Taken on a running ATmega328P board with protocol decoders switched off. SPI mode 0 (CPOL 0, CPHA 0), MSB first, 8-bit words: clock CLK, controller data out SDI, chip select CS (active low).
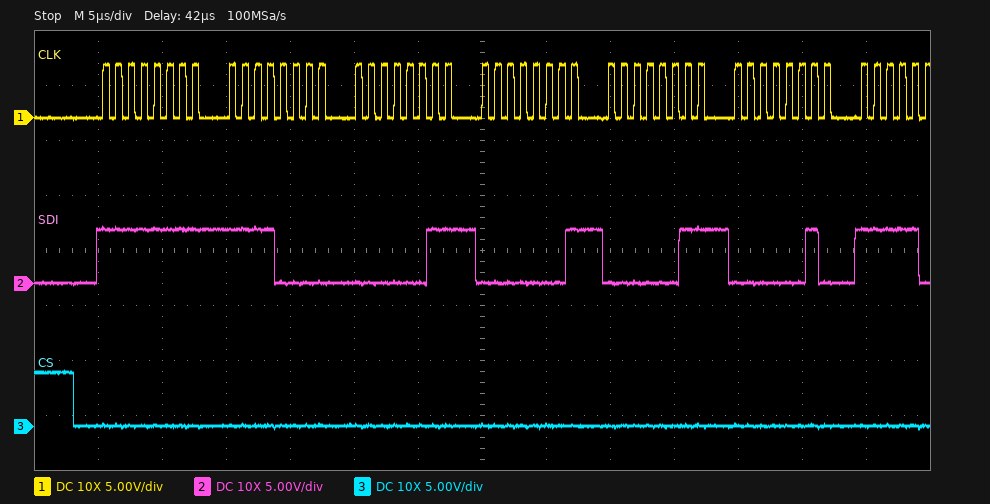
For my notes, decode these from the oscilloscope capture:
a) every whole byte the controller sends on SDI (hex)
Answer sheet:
0xFF 0xF0 0x03 0x01 0x03 0x02
